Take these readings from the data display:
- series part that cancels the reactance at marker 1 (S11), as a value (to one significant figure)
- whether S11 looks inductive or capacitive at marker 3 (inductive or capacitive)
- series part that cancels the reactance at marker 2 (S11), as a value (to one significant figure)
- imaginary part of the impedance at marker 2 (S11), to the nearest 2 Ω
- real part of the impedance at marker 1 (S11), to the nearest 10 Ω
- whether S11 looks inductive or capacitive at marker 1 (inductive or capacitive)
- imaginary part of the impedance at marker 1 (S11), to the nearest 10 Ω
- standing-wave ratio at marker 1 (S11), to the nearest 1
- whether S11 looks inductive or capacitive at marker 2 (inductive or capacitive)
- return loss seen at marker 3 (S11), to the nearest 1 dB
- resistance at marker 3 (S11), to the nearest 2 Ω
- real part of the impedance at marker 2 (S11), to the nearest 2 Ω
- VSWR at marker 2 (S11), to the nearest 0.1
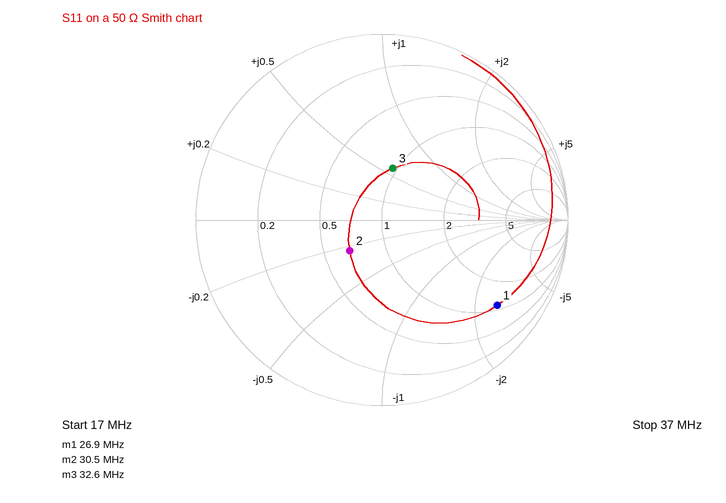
800 nH
inductive
60 nH
-12 Ω
60 Ω
capacitive
-130 Ω
8
capacitive
11 dB
48 Ω
34 Ω
1.6
